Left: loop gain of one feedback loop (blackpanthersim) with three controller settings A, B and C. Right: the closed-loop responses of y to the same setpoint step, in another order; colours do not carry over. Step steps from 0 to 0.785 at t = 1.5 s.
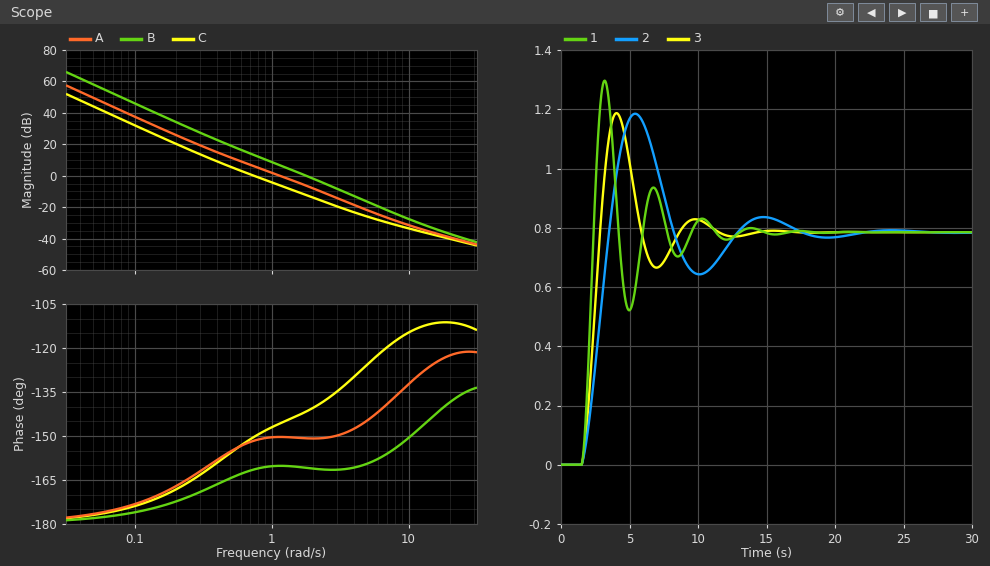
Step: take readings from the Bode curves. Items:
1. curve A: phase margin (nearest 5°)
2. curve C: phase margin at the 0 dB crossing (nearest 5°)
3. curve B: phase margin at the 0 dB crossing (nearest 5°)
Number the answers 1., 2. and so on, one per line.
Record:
1. 30°
2. 30°
3. 20°
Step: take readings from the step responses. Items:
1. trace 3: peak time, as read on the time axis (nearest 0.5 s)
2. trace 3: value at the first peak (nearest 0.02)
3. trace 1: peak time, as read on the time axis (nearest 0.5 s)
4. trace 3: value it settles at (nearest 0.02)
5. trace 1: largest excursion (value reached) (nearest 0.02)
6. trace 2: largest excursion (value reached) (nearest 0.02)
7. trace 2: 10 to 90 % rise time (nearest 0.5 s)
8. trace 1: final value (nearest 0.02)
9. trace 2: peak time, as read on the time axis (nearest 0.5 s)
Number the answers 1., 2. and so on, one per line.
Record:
1. 4.0 s
2. 1.18
3. 3.0 s
4. 0.78
5. 1.30
6. 1.18
7. 1.5 s
8. 0.78
9. 5.5 s
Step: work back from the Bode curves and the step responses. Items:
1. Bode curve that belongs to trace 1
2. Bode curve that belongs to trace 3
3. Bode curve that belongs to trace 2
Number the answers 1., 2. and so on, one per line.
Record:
1. B
2. A
3. C
